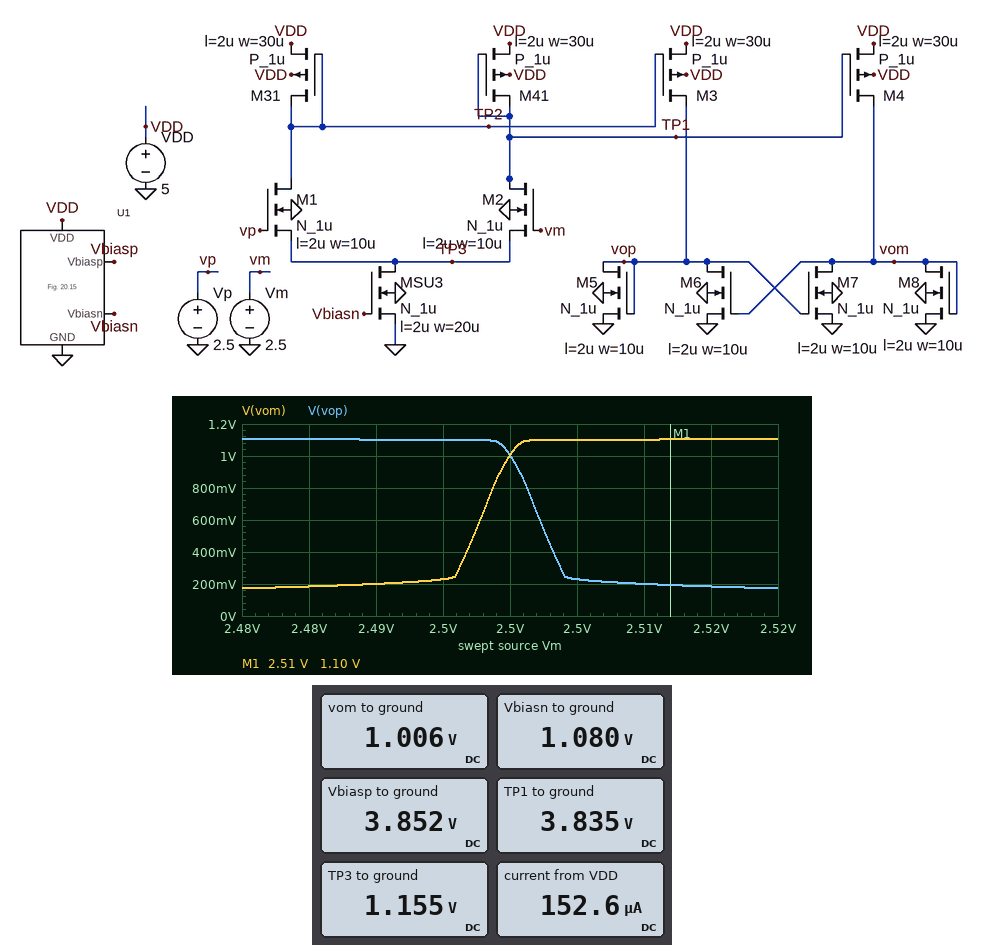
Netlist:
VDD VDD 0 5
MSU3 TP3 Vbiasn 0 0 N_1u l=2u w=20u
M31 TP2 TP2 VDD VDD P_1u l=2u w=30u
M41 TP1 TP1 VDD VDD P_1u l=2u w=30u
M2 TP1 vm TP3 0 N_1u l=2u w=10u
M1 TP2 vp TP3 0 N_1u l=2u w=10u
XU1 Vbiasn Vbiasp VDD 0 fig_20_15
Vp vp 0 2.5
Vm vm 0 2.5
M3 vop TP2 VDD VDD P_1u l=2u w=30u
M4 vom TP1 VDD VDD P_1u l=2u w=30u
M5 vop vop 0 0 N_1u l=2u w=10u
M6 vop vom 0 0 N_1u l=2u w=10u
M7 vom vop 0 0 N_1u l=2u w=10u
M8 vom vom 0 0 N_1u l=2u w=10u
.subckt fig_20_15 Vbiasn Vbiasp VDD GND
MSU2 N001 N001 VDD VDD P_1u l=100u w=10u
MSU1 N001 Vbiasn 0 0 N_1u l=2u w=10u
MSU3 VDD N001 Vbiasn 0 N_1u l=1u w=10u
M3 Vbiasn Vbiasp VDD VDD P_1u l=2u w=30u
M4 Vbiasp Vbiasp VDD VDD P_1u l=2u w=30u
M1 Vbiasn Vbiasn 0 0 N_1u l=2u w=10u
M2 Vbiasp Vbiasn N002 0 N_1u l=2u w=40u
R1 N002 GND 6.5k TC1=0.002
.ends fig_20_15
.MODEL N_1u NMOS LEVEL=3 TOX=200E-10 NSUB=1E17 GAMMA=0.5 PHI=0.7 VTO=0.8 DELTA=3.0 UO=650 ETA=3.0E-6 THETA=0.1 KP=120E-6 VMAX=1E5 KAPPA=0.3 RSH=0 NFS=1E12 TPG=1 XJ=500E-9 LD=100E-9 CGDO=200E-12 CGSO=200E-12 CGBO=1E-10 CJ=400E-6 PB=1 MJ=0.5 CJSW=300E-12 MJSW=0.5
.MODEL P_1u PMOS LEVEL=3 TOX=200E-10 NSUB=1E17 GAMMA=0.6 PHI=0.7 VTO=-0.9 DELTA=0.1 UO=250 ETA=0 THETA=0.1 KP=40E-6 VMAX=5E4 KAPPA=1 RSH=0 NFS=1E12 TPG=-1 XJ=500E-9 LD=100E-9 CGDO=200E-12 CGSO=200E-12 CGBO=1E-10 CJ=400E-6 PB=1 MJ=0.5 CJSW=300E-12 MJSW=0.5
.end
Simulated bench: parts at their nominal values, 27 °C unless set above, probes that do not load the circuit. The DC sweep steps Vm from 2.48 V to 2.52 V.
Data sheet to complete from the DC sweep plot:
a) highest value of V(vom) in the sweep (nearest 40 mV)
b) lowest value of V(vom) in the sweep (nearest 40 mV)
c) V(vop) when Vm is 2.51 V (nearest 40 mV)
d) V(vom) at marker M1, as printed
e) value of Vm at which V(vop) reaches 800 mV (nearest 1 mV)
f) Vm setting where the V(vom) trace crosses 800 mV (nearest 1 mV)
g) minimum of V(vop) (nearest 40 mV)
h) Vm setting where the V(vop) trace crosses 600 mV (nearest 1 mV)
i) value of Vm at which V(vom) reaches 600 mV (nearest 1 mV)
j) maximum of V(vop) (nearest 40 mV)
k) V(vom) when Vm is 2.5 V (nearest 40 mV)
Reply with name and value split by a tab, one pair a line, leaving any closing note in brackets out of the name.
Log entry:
highest value of V(vom) in the sweep	1.12 V
lowest value of V(vom) in the sweep	160 mV
V(vop) when Vm is 2.51 V	200 mV
V(vom) at marker M1, as printed	1.10 V
value of Vm at which V(vop) reaches 800 mV	2.501 V
Vm setting where the V(vom) trace crosses 800 mV	2.499 V
minimum of V(vop)	160 mV
Vm setting where the V(vop) trace crosses 600 mV	2.502 V
value of Vm at which V(vom) reaches 600 mV	2.498 V
maximum of V(vop)	1.12 V
V(vom) when Vm is 2.5 V	1.00 V
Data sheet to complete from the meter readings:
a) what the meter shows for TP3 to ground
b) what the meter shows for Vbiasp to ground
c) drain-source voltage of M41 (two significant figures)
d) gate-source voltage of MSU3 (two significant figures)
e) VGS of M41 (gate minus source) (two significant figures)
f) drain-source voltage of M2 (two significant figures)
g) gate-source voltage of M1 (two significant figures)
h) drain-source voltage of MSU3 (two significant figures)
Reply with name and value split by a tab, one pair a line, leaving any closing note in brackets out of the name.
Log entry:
what the meter shows for TP3 to ground	1.155 V
what the meter shows for Vbiasp to ground	3.852 V
drain-source voltage of M41	-1.2 V
gate-source voltage of MSU3	1.1 V
VGS of M41 (gate minus source)	-1.2 V
drain-source voltage of M2	2.7 V
gate-source voltage of M1	1.3 V
drain-source voltage of MSU3	1.2 V
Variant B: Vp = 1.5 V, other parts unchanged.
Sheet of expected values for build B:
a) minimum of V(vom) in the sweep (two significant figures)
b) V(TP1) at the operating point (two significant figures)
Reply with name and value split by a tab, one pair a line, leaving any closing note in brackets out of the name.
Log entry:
minimum of V(vom) in the sweep	1.2 V
V(TP1) at the operating point	3.7 V
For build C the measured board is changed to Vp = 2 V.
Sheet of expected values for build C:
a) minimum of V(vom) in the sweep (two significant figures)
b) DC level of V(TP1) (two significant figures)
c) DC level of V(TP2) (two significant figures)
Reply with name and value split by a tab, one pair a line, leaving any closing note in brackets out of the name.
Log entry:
minimum of V(vom) in the sweep	1.2 V
DC level of V(TP1)	3.7 V
DC level of V(TP2)	4.2 V
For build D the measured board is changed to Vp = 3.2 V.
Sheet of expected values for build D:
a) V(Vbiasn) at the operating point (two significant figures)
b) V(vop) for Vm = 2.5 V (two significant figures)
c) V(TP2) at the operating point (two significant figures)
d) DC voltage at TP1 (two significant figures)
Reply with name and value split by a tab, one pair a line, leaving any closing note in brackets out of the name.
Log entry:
V(Vbiasn) at the operating point	1.1 V
V(vop) for Vm = 2.5 V	1.2 V
V(TP2) at the operating point	3.7 V
DC voltage at TP1	4.4 V
